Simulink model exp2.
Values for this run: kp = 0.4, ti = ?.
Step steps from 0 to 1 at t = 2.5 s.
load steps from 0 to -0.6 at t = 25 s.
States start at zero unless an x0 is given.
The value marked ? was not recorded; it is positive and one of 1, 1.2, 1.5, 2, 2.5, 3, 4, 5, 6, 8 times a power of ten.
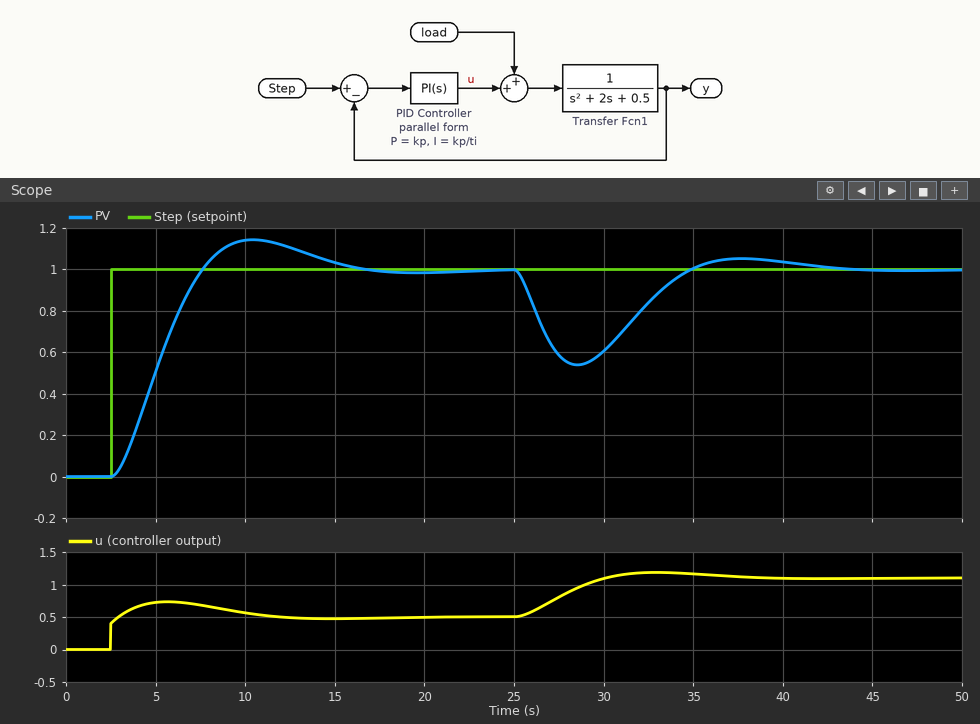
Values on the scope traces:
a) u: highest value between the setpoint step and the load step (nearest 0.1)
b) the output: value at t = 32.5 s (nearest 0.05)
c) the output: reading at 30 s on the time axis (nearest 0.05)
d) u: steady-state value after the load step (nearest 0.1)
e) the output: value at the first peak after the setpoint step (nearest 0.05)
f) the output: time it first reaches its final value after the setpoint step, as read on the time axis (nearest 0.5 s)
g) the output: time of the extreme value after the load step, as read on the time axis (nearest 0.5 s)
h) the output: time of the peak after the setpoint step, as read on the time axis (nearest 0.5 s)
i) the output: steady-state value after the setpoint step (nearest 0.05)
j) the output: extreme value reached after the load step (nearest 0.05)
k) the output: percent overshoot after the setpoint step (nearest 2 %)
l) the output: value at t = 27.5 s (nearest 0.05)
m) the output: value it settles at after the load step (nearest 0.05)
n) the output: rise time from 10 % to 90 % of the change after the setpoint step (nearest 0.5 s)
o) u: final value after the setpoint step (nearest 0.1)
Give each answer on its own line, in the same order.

0.7
0.85
0.60
1.1
1.15
7.5 s
28.5 s
10.5 s
1.00
0.55
14 %
0.60
1.00
3.5 s
0.5
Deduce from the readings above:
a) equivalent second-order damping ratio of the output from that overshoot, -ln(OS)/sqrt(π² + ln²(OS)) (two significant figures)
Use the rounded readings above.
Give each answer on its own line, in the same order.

0.53
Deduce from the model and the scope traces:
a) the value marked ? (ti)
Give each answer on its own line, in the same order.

1.5
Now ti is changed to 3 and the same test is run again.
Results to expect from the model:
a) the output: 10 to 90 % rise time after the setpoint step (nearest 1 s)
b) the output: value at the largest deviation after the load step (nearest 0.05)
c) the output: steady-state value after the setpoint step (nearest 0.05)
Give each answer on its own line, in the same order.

7 s
0.50
1.00
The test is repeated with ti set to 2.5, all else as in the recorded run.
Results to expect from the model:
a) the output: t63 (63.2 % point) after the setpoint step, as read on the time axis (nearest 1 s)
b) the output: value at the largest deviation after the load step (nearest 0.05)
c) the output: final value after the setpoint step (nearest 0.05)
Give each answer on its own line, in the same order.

6 s
0.50
1.00
